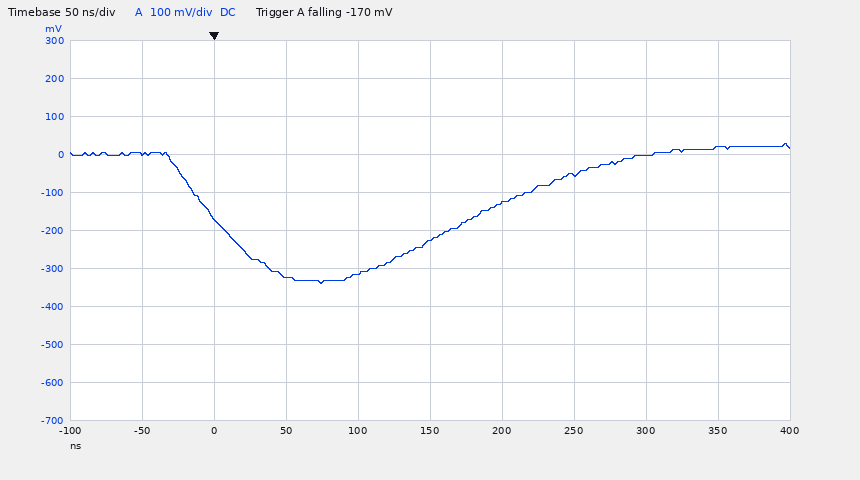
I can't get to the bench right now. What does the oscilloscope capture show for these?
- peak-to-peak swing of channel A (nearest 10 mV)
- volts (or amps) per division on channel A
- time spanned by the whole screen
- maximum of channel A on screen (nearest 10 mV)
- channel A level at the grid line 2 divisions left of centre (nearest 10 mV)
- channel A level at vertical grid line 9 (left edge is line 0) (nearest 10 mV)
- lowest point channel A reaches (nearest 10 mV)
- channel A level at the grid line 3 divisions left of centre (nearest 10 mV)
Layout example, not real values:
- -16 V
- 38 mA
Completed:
- 370 mV
- 100 mV
- 500 ns
- 30 mV
- -320 mV
- 20 mV
- -340 mV
- -170 mV
